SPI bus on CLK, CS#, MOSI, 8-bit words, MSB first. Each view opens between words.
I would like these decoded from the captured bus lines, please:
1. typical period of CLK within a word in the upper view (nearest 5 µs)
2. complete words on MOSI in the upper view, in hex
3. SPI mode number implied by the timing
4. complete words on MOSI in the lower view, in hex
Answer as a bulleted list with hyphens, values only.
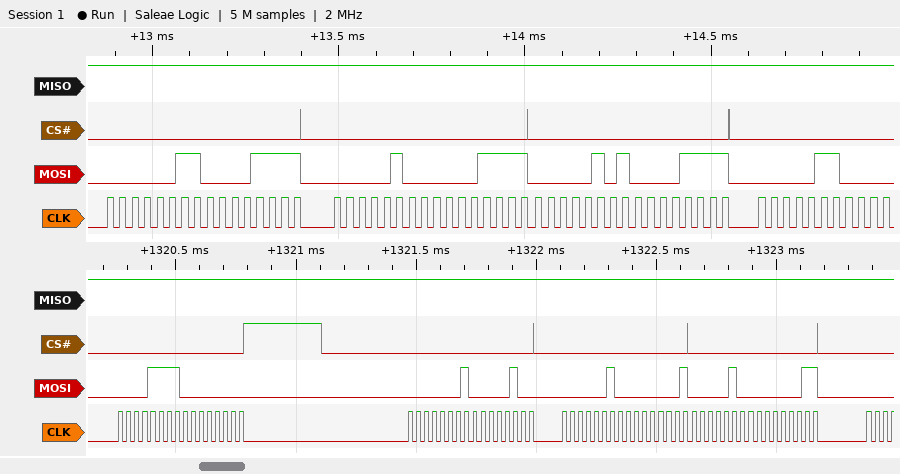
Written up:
- 35 µs
- 03, 0F, 04, 0F, 05, 0F, 06
- 0
- 0F, 00, 01, 04, 02, 01, 04, 03
